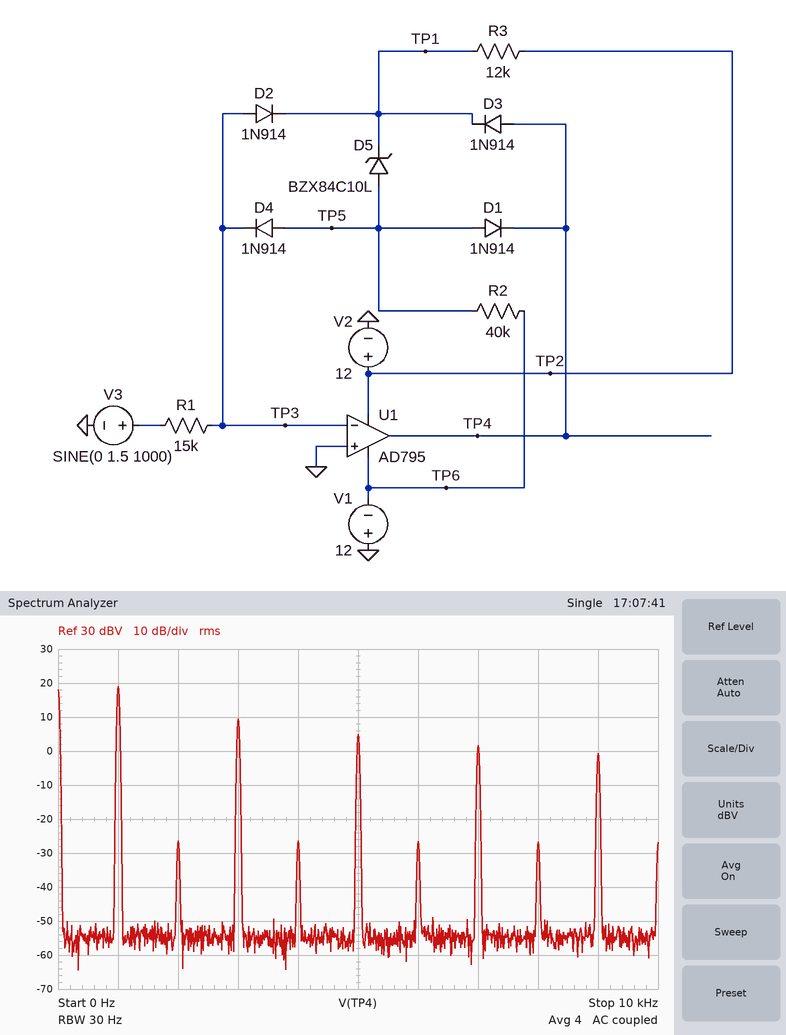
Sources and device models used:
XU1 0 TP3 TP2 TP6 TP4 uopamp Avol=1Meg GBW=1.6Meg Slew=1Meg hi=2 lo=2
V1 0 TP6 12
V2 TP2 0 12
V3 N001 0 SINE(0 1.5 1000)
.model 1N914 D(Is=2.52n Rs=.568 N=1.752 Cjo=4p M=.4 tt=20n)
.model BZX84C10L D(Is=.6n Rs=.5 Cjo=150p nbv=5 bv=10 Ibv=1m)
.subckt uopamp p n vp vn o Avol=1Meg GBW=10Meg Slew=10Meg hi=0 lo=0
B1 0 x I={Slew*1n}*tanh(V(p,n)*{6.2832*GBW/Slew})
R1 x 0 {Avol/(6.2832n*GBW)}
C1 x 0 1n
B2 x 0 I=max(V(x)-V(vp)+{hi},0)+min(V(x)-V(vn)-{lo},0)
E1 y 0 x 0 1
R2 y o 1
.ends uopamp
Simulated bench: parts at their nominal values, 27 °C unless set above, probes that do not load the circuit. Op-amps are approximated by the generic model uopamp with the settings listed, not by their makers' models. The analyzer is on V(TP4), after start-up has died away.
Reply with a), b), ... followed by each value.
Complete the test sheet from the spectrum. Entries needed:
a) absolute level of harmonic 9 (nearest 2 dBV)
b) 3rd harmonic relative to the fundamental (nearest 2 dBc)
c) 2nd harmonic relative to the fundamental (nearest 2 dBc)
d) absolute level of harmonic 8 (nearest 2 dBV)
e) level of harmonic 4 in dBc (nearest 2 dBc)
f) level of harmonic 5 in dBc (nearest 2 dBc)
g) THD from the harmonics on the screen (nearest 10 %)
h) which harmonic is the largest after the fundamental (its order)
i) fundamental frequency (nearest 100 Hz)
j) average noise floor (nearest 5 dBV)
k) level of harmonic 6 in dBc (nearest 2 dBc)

a) 0 dBV
b) -10 dBc
c) -46 dBc
d) -26 dBV
e) -46 dBc
f) -14 dBc
g) 40 %
h) 3
i) 1.0 kHz
j) -55 dBV
k) -46 dBc
